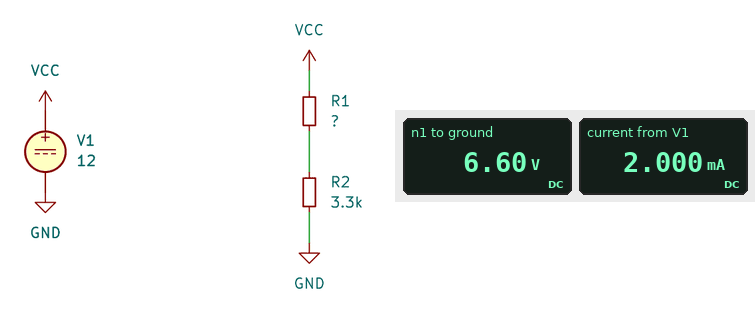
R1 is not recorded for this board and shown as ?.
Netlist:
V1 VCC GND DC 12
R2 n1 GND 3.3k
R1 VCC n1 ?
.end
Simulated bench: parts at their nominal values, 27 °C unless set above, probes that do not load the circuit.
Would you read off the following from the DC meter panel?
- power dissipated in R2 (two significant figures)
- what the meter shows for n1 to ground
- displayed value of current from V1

13 mW
6.60 V
2.000 mA
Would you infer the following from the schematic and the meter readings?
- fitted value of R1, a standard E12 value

2.7 kΩ
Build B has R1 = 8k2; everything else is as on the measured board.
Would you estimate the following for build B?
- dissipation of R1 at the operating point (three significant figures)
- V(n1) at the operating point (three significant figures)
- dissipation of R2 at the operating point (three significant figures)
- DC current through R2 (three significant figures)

8.93 mW
3.44 V
3.59 mW
1.04 mA
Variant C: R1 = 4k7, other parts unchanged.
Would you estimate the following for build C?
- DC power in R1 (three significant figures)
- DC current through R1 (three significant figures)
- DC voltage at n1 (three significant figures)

10.6 mW
1.50 mA
4.95 V
